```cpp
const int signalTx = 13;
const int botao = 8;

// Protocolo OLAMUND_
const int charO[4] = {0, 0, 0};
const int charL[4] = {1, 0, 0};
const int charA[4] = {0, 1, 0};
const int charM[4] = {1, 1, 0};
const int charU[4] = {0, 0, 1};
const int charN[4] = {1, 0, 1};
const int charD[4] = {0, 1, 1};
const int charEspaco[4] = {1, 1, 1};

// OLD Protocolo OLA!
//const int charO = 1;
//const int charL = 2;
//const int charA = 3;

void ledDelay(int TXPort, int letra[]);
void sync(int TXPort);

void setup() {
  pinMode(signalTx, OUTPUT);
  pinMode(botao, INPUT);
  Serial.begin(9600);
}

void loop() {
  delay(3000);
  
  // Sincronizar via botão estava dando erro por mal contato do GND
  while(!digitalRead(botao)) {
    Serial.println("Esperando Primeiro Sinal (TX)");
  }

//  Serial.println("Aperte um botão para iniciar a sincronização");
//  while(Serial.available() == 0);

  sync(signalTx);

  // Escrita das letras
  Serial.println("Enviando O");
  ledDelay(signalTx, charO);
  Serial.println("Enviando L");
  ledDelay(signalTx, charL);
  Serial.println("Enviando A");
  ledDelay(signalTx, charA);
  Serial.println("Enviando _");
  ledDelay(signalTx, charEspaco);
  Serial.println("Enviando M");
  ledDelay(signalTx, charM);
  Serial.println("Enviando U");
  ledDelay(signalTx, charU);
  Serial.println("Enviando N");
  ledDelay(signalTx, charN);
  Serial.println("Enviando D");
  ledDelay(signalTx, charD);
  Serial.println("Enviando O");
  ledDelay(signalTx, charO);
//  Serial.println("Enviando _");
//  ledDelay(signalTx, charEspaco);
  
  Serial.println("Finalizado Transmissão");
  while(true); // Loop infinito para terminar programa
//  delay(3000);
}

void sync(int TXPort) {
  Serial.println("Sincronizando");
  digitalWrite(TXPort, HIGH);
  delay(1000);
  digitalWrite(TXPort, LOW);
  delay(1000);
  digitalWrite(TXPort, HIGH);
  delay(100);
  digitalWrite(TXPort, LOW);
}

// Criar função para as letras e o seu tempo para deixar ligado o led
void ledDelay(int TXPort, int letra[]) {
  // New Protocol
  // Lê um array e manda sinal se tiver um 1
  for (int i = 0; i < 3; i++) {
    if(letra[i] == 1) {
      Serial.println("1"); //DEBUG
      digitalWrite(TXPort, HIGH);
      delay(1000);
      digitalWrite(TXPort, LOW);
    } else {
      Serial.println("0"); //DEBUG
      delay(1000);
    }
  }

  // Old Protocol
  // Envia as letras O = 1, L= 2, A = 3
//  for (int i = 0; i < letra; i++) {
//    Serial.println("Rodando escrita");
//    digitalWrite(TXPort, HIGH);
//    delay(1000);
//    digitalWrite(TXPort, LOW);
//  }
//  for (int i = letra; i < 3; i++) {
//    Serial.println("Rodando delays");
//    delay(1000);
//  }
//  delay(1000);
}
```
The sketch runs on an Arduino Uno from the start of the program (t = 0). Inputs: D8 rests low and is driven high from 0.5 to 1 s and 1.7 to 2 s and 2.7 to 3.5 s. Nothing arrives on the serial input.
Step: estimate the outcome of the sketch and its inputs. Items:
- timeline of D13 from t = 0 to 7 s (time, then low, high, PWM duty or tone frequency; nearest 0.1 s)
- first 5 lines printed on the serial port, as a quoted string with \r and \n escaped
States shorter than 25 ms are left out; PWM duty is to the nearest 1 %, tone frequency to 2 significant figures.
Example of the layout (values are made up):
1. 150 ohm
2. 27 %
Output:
1. 0 s low; 3 s high; 4 s low; 5 s high; 5.1 s low
2. "Sincronizando\r\nEnviando O\r\n0\r\n0\r\n0\r\n"
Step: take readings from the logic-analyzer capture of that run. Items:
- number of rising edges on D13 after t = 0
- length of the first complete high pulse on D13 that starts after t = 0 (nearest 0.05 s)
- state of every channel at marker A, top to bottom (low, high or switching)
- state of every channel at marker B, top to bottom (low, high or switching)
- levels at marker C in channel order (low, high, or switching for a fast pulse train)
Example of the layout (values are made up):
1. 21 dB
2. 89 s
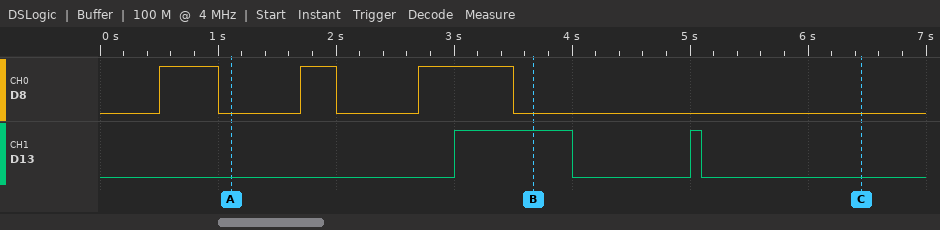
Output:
1. 2
2. 1.00 s
3. D8 low, D13 low
4. D8 low, D13 high
5. D8 low, D13 low
